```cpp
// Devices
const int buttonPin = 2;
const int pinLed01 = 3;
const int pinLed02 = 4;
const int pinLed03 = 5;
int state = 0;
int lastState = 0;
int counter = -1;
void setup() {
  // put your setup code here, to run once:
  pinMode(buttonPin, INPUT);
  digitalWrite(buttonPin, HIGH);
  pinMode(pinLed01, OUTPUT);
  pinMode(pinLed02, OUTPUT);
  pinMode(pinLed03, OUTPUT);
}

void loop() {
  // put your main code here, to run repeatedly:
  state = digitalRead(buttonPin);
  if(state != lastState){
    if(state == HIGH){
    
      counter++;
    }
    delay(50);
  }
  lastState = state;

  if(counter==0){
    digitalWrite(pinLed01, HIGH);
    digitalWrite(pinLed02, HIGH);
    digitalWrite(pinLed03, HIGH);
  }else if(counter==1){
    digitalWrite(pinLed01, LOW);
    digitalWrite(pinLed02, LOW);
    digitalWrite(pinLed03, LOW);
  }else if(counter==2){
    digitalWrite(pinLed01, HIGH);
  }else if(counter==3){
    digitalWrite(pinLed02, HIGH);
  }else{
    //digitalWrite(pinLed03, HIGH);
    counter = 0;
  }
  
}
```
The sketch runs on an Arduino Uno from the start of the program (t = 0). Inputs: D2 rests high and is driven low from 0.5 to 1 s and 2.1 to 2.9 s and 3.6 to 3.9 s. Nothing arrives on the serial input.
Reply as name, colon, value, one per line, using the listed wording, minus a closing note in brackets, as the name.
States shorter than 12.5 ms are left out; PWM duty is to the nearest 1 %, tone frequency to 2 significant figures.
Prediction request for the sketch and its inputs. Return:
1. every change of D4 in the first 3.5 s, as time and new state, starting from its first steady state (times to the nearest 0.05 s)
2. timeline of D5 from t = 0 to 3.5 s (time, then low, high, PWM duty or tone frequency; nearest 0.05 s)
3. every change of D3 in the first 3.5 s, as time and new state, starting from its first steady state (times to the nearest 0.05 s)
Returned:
every change of D4 in the first 3.5 s, as time and new state, starting from its first steady state: 0 s low; 0.05 s high; 1.05 s low
timeline of D5 from t = 0 to 3.5 s: 0 s low; 0.05 s high; 1.05 s low
every change of D3 in the first 3.5 s, as time and new state, starting from its first steady state: 0 s low; 0.05 s high; 1.05 s low; 2.95 s high
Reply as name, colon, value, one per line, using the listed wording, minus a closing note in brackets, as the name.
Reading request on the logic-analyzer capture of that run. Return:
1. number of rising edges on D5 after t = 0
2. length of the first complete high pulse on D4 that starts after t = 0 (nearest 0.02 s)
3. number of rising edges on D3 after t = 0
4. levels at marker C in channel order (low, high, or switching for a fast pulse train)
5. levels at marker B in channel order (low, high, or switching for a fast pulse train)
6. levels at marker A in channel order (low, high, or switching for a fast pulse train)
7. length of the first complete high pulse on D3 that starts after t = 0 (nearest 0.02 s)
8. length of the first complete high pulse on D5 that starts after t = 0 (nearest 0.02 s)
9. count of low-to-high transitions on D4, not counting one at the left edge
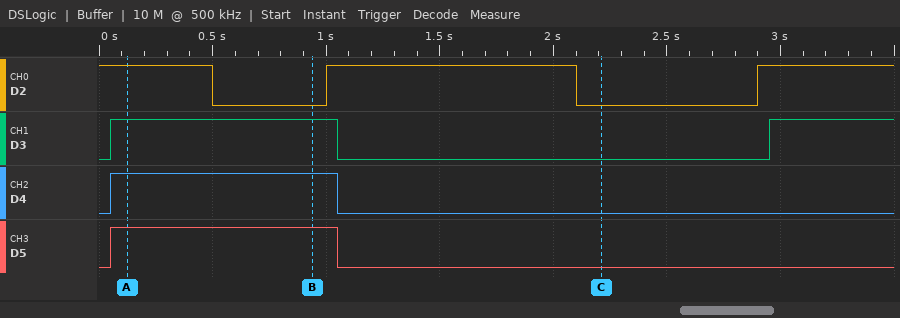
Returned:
number of rising edges on D5 after t = 0: 1
length of the first complete high pulse on D4 that starts after t = 0: 1.00 s
number of rising edges on D3 after t = 0: 2
levels at marker C in channel order: D2 low, D3 low, D4 low, D5 low
levels at marker B in channel order: D2 low, D3 high, D4 high, D5 high
levels at marker A in channel order: D2 high, D3 high, D4 high, D5 high
length of the first complete high pulse on D3 that starts after t = 0: 1.00 s
length of the first complete high pulse on D5 that starts after t = 0: 1.00 s
count of low-to-high transitions on D4, not counting one at the left edge: 1
